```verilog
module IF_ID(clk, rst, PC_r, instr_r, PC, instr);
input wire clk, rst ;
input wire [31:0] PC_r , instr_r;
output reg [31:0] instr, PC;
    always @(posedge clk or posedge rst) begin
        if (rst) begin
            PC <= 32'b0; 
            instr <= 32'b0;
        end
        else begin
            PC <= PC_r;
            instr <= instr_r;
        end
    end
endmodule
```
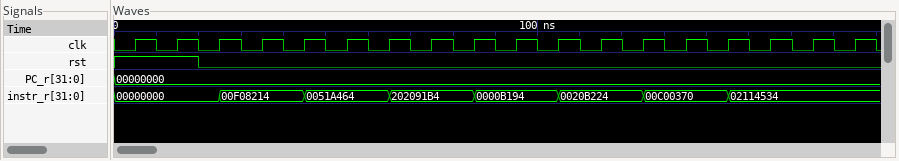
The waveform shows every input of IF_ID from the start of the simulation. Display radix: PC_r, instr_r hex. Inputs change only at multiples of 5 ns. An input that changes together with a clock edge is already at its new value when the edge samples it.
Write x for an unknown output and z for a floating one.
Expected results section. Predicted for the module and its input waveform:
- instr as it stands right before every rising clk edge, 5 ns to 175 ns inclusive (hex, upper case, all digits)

00000000, 00000000, 00000000, 00F08214, 00F08214, 0051A464, 0051A464, 202091B4, 202091B4, 0000B194, 0000B194, 0020B224, 0020B224, 00C00370, 00C00370, 02114534, 02114534, 02114534
